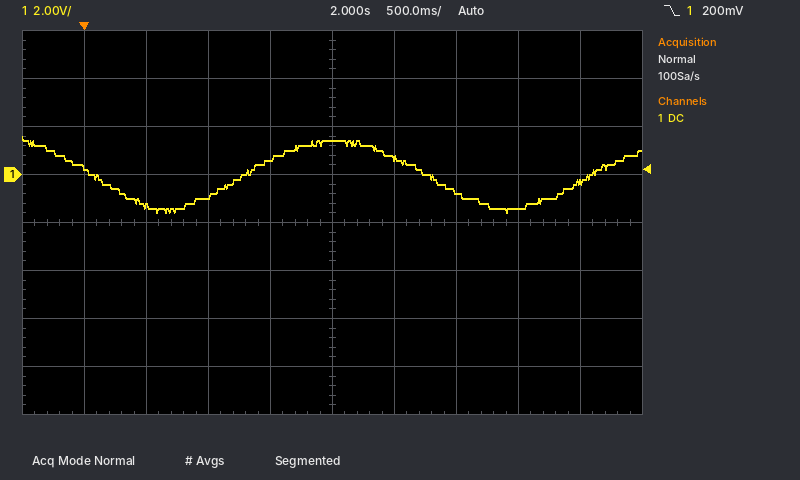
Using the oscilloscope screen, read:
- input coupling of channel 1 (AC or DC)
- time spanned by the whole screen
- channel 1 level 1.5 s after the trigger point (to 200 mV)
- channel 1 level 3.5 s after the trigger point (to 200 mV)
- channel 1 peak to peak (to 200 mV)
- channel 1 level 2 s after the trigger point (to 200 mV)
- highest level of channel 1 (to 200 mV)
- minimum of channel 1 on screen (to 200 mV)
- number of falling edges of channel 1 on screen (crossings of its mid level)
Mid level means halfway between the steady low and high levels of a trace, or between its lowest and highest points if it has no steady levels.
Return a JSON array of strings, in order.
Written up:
["DC", "5 s", "600 mV", "-1.4 V", "3.2 V", "1.4 V", "1.6 V", "-1.6 V", "2"]
